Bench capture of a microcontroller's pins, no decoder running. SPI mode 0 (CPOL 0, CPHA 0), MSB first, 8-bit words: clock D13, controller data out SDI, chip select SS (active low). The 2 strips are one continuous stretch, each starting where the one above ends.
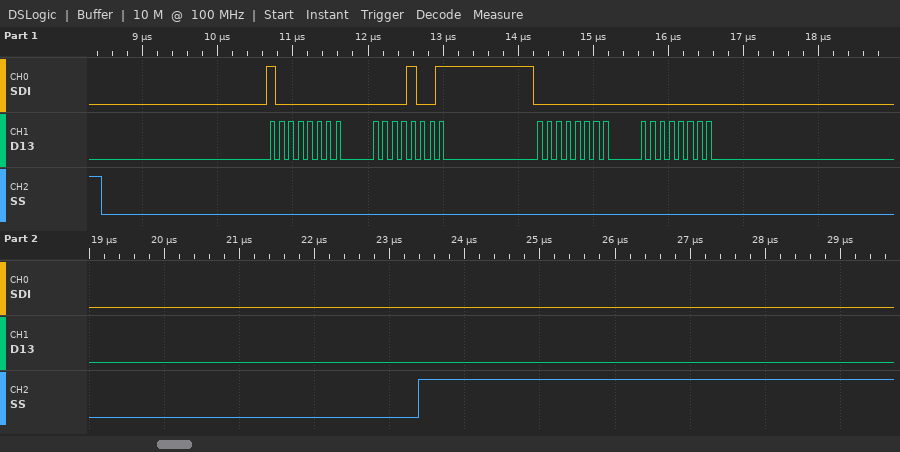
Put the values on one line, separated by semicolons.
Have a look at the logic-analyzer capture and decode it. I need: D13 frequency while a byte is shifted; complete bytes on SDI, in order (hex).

8 MHz; 80 09 00 00
